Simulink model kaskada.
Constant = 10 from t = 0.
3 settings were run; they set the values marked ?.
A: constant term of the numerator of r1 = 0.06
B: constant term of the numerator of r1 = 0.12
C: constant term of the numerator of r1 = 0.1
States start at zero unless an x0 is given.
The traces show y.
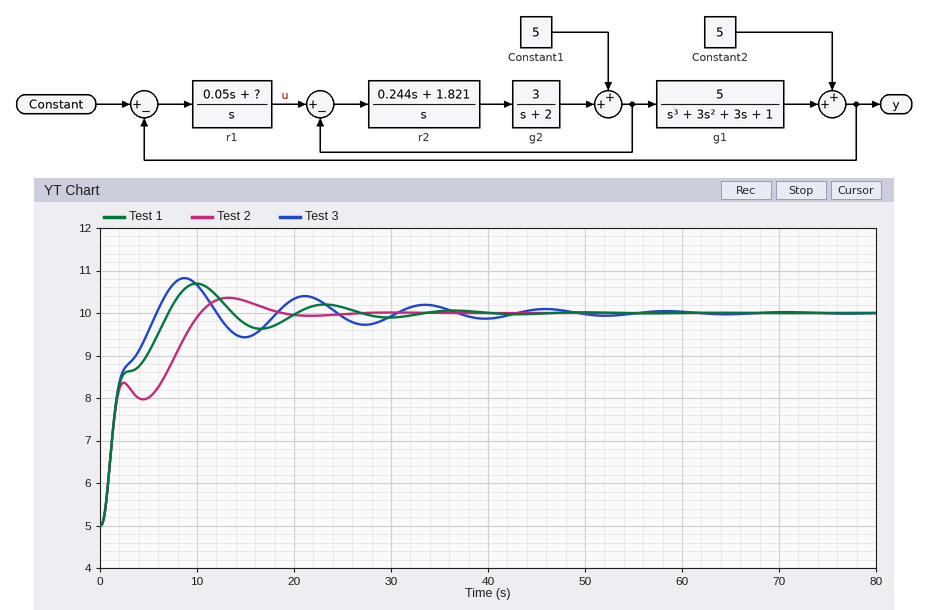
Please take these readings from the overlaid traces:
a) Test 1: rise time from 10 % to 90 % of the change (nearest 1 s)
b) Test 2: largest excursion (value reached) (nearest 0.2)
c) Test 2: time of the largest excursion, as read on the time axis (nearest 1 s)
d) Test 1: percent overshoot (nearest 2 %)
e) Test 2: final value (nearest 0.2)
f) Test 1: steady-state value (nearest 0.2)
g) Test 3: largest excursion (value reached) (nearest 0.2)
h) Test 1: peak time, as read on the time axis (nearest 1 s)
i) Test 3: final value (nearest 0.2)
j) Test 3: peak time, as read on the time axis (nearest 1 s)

5 s
10.4
13 s
14 %
10.0
10.0
10.8
10 s
10.0
9 s
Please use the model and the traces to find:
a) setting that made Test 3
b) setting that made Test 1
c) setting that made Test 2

B
C
A
